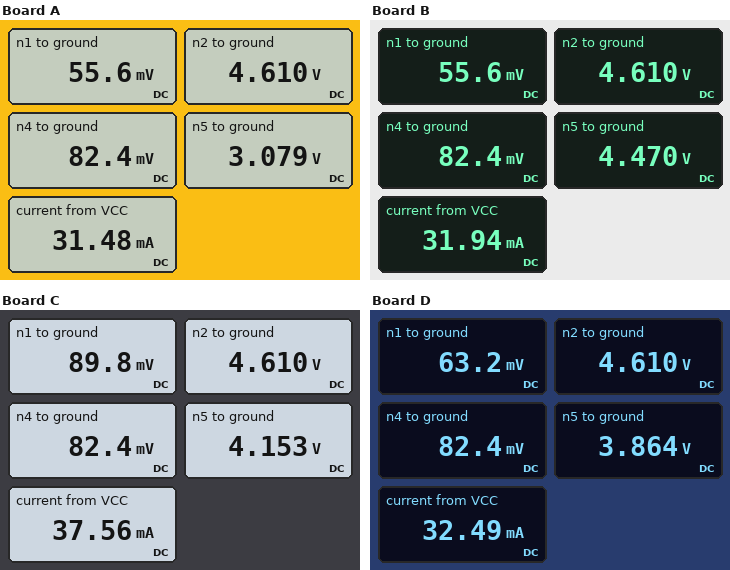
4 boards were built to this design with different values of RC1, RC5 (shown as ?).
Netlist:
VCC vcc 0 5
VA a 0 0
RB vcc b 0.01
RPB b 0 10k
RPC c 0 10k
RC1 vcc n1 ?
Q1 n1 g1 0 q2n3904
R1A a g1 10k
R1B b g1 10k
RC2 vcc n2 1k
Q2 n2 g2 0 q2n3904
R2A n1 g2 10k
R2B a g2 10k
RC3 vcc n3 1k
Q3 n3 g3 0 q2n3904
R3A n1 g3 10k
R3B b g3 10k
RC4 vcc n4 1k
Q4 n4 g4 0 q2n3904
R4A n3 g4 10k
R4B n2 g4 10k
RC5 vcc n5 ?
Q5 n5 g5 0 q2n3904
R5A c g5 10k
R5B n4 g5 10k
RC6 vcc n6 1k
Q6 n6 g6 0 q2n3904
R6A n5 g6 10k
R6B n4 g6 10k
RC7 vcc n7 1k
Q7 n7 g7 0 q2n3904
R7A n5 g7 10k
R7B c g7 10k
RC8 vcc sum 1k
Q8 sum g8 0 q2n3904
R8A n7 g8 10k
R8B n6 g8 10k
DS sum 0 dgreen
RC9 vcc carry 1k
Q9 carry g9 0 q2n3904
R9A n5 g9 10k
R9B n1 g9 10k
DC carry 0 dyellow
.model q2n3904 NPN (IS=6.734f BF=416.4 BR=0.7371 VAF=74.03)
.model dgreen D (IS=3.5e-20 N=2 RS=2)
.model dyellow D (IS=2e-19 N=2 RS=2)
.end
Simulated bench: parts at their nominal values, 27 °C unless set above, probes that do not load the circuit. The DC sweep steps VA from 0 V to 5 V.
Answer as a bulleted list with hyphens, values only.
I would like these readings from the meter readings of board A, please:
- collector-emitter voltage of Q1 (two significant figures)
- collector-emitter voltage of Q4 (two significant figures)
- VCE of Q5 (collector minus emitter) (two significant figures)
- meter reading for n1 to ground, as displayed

- 56 mV
- 82 mV
- 3.1 V
- 55.6 mV
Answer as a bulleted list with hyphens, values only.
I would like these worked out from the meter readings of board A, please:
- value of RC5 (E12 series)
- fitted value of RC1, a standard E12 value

- 2.7 kΩ
- 3.3 kΩ
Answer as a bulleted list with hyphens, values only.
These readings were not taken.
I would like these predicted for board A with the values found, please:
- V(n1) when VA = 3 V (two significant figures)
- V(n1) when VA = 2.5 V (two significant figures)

- 45 mV
- 47 mV
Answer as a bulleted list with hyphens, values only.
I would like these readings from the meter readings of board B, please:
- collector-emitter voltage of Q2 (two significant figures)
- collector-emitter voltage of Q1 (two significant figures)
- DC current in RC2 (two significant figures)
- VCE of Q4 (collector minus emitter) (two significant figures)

- 4.6 V
- 56 mV
- 390 µA
- 82 mV
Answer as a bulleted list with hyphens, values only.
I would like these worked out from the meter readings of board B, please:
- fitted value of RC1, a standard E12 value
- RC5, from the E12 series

- 3.3 kΩ
- 470 Ω
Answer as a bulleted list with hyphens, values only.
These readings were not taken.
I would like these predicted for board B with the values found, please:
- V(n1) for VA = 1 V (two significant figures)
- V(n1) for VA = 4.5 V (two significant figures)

- 52 mV
- 42 mV
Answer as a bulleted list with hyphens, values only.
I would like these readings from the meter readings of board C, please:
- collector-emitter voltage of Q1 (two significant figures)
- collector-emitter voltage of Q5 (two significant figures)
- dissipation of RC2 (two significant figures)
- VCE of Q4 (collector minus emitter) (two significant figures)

- 90 mV
- 4.2 V
- 150 µW
- 82 mV
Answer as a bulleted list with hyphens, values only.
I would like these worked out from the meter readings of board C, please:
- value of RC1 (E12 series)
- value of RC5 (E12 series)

- 680 Ω
- 820 Ω
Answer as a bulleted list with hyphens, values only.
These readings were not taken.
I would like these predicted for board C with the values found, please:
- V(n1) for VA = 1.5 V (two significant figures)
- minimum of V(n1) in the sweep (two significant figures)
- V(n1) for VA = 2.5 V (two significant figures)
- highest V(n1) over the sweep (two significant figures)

- 81 mV
- 69 mV
- 77 mV
- 90 mV
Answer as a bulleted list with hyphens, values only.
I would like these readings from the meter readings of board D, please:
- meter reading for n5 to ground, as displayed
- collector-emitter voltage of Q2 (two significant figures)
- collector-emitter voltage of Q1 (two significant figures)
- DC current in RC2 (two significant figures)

- 3.864 V
- 4.6 V
- 63 mV
- 390 µA
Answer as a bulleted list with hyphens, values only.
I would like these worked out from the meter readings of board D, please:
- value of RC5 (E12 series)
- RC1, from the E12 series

- 1.2 kΩ
- 2.2 kΩ
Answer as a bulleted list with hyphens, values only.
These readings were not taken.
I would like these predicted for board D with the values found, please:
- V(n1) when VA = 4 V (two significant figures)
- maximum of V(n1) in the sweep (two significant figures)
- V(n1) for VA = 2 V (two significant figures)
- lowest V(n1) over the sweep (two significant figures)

- 49 mV
- 63 mV
- 55 mV
- 47 mV
